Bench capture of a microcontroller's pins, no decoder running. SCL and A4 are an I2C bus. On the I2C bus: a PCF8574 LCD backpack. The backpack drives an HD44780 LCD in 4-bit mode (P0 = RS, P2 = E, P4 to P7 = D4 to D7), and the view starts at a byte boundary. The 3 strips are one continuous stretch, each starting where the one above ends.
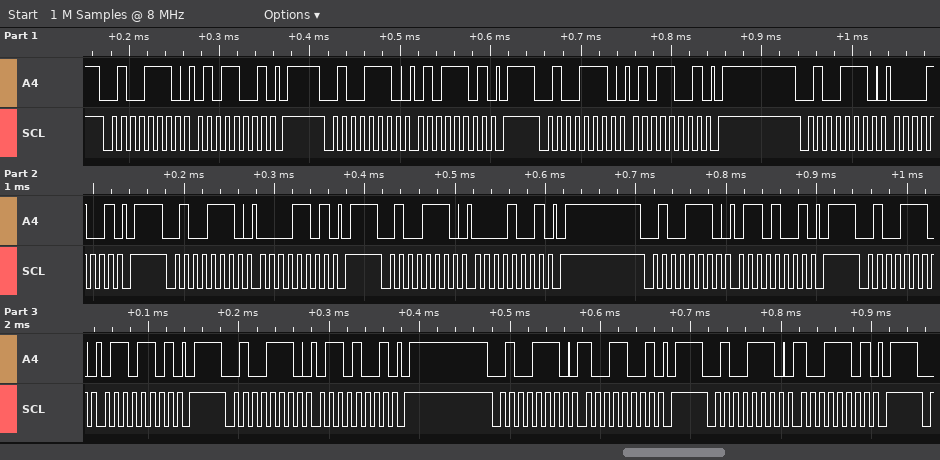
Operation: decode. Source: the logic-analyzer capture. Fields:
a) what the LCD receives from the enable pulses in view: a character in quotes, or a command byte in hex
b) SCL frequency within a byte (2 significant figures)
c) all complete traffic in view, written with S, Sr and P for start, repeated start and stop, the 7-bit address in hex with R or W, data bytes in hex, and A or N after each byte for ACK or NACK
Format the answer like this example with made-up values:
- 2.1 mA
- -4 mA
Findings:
- 'P'
- 100 kHz
- S 27W A 59 A P S 27W A 5D A P S 27W A 59 A P S 27W A 09 A P S 27W A 0D A P S 27W A 09 A P S 27W A 69 A P S 27W A 6D A P S 27W A 69 A P S 27W A 99 A P S 27W A 9D A P
